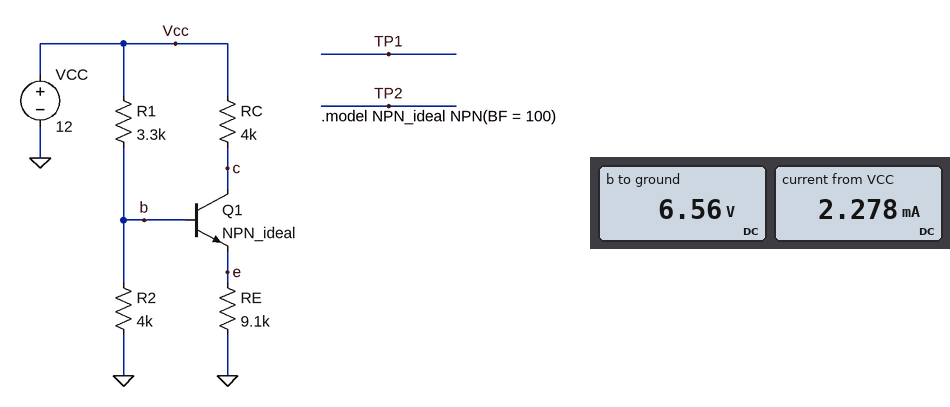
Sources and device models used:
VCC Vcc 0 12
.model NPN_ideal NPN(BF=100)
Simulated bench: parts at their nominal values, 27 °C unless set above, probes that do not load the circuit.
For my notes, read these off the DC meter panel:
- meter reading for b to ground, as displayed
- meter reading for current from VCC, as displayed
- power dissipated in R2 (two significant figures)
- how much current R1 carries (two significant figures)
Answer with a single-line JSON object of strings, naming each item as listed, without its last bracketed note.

{"meter reading for b to ground, as displayed": "6.56 V", "meter reading for current from VCC, as displayed": "2.278 mA", "power dissipated in R2": "11 mW", "how much current R1 carries": "1.6 mA"}
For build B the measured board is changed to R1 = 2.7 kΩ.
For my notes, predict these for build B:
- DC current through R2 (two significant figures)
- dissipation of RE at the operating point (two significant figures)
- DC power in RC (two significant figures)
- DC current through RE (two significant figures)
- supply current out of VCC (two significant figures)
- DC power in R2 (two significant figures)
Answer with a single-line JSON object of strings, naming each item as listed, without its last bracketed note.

{"DC current through R2": "1.8 mA", "dissipation of RE at the operating point": "4.5 mW", "DC power in RC": "1.9 mW", "DC current through RE": "700 µA", "supply current out of VCC": "2.5 mA", "DC power in R2": "13 mW"}
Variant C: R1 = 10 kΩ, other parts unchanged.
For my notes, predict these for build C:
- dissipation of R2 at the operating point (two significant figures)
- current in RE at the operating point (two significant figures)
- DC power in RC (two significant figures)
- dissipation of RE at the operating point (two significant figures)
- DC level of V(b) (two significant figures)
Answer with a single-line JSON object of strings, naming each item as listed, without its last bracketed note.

{"dissipation of R2 at the operating point": "2.9 mW", "current in RE at the operating point": "290 µA", "DC power in RC": "340 µW", "dissipation of RE at the operating point": "790 µW", "DC level of V(b)": "3.4 V"}
